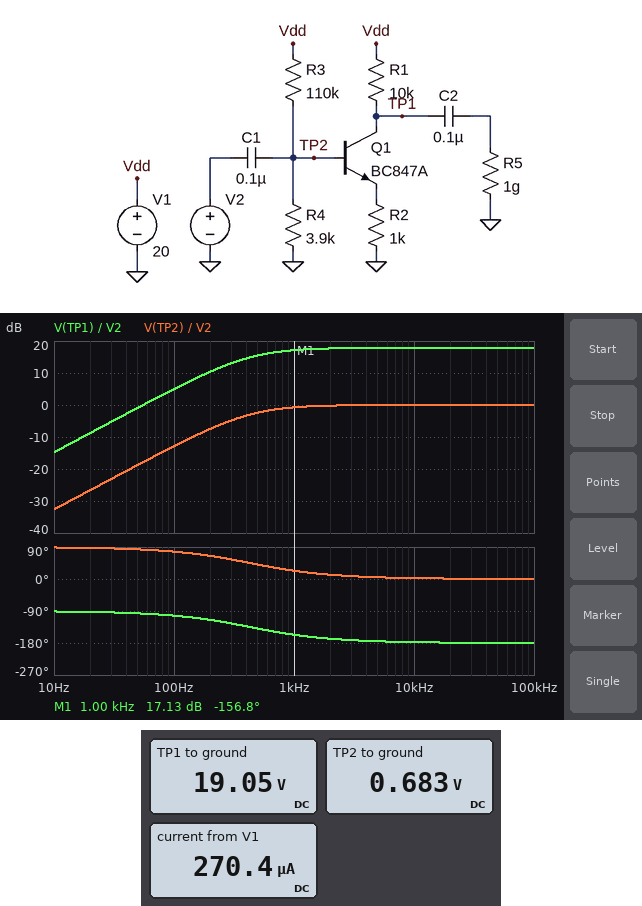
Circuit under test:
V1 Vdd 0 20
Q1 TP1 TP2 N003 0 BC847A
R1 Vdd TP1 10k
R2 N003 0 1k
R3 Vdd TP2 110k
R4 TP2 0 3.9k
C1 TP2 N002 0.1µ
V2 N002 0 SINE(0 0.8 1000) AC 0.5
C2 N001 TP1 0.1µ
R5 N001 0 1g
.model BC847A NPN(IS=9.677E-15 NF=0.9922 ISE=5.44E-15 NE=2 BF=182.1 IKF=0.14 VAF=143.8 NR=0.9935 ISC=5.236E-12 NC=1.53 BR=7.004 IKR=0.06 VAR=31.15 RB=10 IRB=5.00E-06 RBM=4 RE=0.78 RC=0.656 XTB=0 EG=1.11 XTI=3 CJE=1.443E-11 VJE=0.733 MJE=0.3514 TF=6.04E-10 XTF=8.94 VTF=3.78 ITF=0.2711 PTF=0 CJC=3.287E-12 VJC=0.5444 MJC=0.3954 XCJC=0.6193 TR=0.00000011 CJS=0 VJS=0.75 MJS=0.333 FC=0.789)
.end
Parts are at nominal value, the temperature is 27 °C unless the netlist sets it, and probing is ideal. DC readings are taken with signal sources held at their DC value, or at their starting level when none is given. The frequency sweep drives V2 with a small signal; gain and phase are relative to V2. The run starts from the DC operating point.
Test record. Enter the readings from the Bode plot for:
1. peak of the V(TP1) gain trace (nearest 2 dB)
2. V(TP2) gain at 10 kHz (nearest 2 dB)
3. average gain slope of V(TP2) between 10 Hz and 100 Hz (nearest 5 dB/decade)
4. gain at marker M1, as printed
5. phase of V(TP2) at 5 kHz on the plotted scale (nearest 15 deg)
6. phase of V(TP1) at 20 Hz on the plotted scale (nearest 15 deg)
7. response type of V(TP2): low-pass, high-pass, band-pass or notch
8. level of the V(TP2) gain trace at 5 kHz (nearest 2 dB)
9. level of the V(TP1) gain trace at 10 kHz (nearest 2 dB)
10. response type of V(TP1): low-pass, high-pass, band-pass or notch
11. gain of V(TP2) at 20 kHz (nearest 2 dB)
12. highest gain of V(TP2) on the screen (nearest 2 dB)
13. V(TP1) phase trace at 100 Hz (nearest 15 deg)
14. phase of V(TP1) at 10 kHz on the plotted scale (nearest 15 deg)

18 dB
0 dB
20 dB/decade
17.13 dB
0 deg
-90 deg
high-pass
0 dB
18 dB
high-pass
0 dB
0 dB
-105 deg
-180 deg
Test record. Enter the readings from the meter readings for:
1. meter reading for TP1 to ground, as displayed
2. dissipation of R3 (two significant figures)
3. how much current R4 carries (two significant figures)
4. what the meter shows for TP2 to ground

19.05 V
3.4 mW
180 µA
0.683 V
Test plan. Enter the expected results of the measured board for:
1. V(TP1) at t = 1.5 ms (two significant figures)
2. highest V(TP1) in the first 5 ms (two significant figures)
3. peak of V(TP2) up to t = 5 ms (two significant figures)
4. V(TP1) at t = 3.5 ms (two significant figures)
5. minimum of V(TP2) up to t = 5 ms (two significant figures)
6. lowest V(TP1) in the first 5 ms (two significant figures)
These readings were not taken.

20 V
20 V
1.4 V
20 V
-100 mV
12 V
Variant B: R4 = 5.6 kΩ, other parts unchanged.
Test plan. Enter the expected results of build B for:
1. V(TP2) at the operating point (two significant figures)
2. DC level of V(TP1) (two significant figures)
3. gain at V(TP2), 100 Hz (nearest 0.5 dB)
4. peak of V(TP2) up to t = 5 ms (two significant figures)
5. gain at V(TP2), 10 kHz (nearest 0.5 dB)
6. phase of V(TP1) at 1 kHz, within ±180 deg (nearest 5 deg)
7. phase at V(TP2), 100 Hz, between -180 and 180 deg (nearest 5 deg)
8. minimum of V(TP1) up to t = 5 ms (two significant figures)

960 mV
17 V
-10.0 dB
1.7 V
0 dB
-165 deg
70 deg
9.4 V
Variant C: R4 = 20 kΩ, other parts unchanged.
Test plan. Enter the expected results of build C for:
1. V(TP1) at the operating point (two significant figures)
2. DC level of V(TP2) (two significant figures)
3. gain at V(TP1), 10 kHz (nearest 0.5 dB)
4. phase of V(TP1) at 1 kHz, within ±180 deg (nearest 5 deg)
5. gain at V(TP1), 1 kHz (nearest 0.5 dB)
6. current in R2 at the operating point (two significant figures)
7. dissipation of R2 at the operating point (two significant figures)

1.9 V
2.5 V
-11.5 dB
-125 deg
-17.0 dB
1.8 mA
3.4 mW
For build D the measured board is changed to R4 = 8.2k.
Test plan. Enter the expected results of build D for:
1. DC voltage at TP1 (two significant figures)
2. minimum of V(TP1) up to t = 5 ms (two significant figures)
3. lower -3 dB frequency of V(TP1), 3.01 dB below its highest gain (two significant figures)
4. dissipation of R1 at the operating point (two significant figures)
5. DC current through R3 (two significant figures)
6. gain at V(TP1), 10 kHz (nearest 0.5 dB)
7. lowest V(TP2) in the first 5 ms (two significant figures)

13 V
5.3 V
220 Hz
5.1 mW
170 µA
19.5 dB
510 mV
